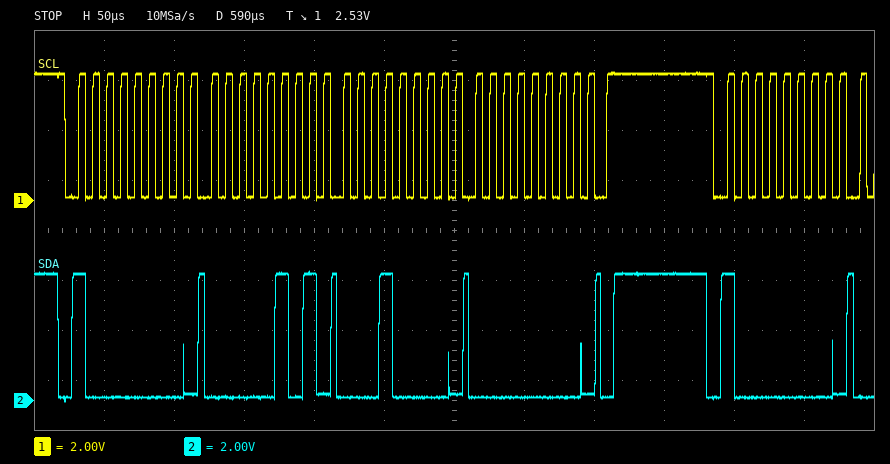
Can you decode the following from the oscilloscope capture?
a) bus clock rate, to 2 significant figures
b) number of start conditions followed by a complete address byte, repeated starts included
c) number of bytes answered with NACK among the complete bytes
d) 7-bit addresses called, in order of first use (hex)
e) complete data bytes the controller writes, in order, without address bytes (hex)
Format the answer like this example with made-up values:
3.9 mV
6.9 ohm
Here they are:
100 kHz
2
0
0x40
05 10 00
